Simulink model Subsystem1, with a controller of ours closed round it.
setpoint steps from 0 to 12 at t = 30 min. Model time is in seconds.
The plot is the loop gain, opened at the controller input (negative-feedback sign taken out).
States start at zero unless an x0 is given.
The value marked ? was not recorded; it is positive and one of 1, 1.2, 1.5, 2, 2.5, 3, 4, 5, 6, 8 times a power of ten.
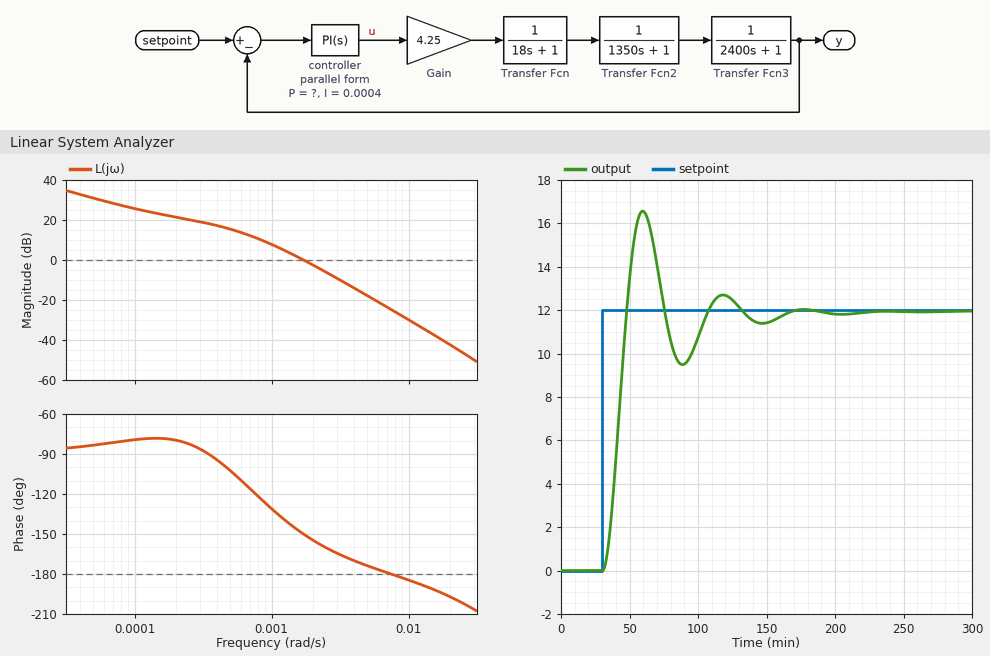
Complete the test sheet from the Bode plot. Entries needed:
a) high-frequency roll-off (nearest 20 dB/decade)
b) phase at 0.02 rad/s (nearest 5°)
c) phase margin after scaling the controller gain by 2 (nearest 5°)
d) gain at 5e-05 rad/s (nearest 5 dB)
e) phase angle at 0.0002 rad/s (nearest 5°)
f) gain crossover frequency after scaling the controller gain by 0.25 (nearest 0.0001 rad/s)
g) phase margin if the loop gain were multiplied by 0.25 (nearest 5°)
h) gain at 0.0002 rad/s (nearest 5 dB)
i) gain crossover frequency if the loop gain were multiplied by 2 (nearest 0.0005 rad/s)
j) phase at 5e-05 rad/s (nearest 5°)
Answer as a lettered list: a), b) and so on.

a) -40 dB/decade
b) -195°
c) 20°
d) 30 dB
e) -80°
f) 0.0007 rad/s
g) 65°
h) 20 dB
i) 0.0025 rad/s
j) -85°
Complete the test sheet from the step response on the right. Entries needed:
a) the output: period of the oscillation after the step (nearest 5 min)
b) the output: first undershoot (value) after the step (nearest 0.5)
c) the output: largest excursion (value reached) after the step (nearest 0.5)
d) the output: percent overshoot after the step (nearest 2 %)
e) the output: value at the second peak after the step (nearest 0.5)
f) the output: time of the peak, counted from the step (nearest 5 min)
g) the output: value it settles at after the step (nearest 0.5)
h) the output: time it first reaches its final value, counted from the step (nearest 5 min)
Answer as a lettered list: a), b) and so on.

a) 60 min
b) 9.5
c) 16.5
d) 38 %
e) 12.5
f) 30 min
g) 12.0
h) 20 min
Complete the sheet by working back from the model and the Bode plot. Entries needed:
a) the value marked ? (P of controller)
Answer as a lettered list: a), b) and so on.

a) 2.5
